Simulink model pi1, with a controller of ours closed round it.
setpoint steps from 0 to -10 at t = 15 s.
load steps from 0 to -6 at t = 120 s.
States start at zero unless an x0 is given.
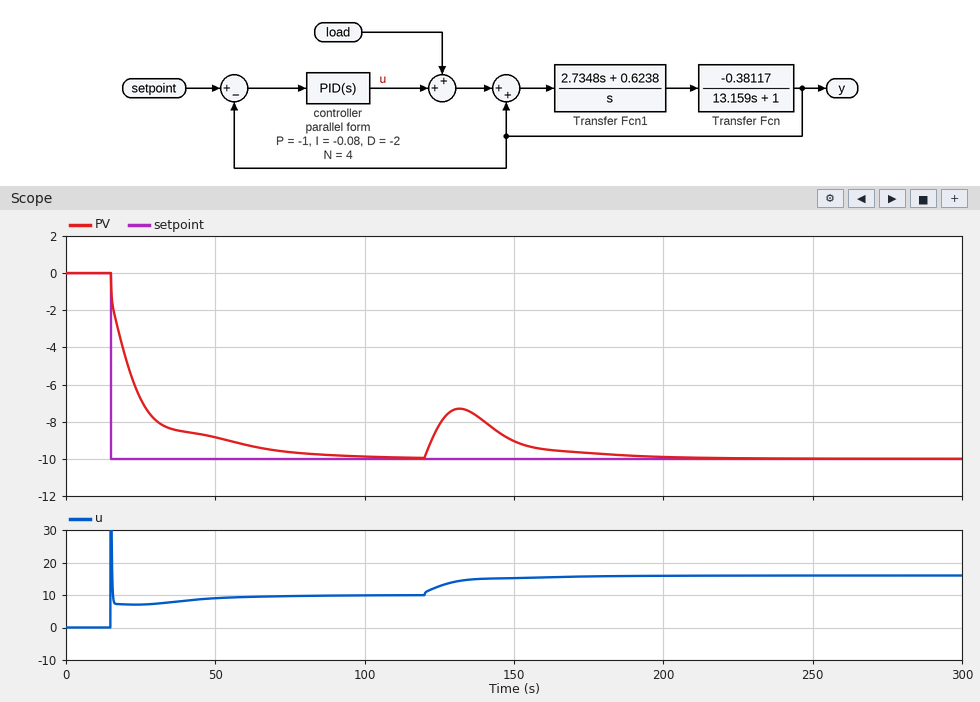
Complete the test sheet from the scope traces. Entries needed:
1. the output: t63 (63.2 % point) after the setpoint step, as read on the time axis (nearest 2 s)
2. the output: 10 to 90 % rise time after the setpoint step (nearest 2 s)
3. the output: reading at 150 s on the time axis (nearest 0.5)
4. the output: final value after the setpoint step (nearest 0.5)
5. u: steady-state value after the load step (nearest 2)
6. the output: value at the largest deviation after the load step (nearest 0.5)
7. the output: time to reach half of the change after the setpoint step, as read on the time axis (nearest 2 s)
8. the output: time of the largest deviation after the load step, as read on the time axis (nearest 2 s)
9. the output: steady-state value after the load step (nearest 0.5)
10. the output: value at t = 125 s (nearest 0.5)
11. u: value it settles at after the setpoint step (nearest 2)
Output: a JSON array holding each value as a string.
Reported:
["24 s", "38 s", "-9.0", "-10.0", "16", "-7.5", "20 s", "132 s", "-10.0", "-8.0", "10"]
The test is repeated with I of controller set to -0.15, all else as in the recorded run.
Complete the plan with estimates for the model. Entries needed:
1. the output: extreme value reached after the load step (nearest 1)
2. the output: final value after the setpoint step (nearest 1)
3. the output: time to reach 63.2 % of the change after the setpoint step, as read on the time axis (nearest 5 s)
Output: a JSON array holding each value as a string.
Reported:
["-8", "-10", "20 s"]
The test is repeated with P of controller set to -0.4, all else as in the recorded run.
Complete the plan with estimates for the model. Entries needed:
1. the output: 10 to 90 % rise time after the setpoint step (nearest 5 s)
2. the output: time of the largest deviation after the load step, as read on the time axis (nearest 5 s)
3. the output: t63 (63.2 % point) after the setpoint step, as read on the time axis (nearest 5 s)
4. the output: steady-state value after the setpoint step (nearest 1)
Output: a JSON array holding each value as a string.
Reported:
["25 s", "135 s", "30 s", "-10"]
